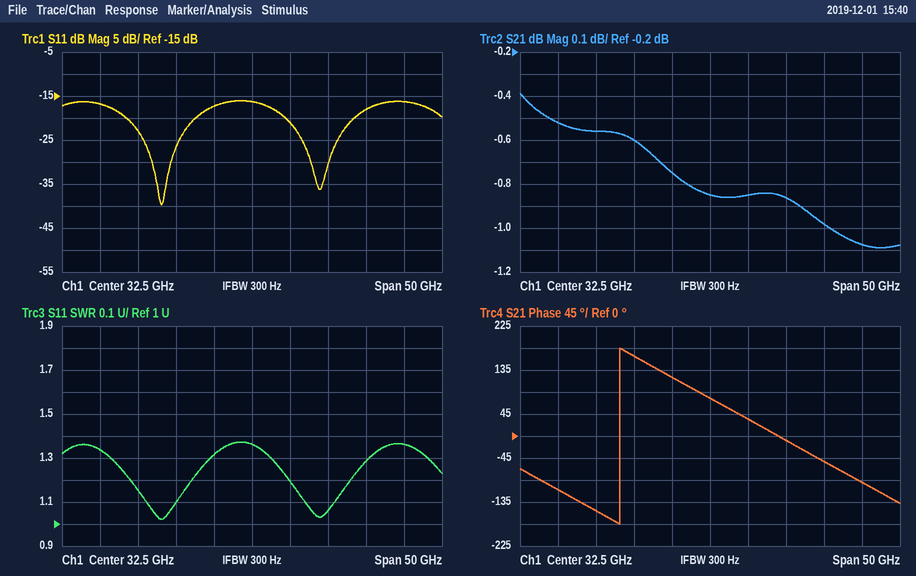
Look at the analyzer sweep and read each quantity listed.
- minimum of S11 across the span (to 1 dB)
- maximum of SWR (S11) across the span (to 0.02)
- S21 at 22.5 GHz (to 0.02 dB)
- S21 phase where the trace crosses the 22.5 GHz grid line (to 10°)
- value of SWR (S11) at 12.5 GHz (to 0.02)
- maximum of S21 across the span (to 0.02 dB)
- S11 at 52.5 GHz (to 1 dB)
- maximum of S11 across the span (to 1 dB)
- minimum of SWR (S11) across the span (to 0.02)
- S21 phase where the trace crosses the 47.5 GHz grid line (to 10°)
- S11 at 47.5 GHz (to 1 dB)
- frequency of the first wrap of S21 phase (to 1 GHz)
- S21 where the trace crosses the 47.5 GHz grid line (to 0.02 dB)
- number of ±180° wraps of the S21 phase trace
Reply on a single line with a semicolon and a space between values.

-40 dB; 1.38; -0.60 dB; 160°; 1.34; -0.38 dB; -16 dB; -16 dB; 1.02; -50°; -18 dB; 21 GHz; -0.98 dB; 1
